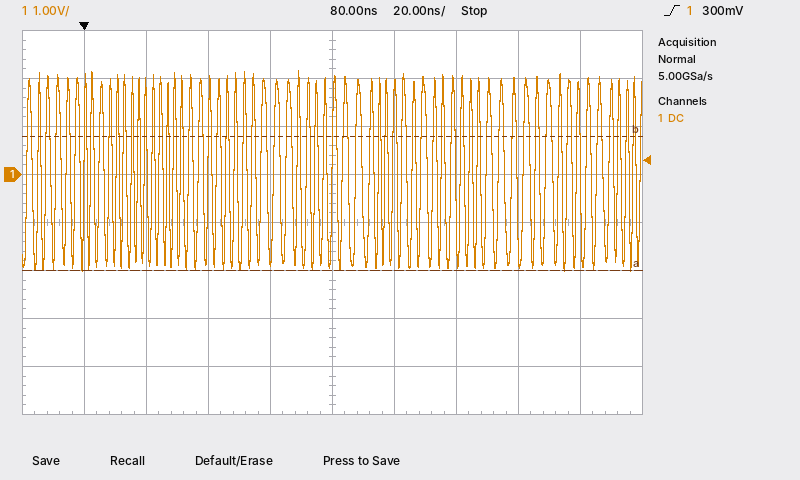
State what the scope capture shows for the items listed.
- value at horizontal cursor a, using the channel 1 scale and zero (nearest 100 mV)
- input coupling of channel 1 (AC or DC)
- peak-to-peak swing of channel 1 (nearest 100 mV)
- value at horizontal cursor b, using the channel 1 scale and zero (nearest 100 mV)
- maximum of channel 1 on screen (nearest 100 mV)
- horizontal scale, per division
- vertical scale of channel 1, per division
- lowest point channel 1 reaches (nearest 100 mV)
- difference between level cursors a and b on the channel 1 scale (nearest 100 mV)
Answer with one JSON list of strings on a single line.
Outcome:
["-2.0 V", "DC", "4.2 V", "800 mV", "2.2 V", "20 ns", "1 V", "-2.0 V", "2.8 V"]
